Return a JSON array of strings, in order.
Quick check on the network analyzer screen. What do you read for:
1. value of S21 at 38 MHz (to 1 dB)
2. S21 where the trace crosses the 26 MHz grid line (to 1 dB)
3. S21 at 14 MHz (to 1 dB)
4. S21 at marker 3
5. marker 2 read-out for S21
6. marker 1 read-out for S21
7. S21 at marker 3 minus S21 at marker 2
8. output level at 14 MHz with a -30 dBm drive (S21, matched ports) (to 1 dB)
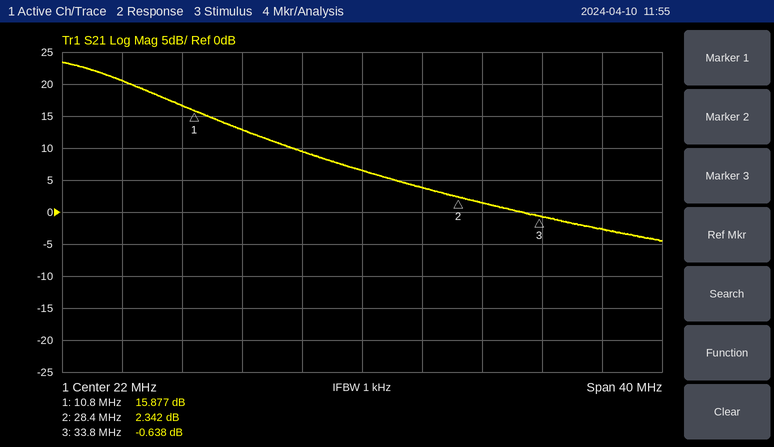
["-3 dB", "4 dB", "13 dB", "-0.638 dB", "2.342 dB", "15.877 dB", "-2.980 dB", "-17 dBm"]
